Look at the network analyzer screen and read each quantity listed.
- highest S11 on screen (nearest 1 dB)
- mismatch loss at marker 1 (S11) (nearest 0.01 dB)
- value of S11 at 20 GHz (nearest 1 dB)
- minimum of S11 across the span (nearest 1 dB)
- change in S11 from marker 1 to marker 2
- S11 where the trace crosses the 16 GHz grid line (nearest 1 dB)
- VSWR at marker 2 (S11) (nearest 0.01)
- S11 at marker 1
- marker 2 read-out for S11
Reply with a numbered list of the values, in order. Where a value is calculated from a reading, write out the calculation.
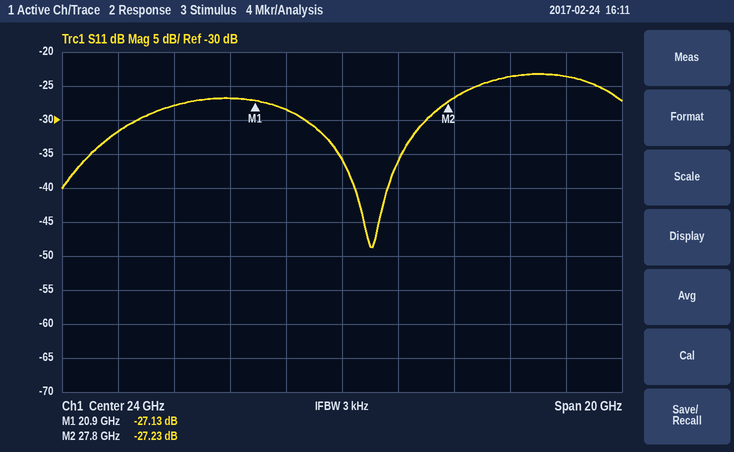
1. -23 dB
2. −10 log10(1 − 10^(-27.13/10)) ≈ 0.01 dB
3. -27 dB
4. -49 dB
5. -27.23 − (-27.13) = -0.10 dB
6. -32 dB
7. (1 + 0.0435)/(1 − 0.0435) ≈ 1.09
8. -27.13 dB
9. -27.23 dB
